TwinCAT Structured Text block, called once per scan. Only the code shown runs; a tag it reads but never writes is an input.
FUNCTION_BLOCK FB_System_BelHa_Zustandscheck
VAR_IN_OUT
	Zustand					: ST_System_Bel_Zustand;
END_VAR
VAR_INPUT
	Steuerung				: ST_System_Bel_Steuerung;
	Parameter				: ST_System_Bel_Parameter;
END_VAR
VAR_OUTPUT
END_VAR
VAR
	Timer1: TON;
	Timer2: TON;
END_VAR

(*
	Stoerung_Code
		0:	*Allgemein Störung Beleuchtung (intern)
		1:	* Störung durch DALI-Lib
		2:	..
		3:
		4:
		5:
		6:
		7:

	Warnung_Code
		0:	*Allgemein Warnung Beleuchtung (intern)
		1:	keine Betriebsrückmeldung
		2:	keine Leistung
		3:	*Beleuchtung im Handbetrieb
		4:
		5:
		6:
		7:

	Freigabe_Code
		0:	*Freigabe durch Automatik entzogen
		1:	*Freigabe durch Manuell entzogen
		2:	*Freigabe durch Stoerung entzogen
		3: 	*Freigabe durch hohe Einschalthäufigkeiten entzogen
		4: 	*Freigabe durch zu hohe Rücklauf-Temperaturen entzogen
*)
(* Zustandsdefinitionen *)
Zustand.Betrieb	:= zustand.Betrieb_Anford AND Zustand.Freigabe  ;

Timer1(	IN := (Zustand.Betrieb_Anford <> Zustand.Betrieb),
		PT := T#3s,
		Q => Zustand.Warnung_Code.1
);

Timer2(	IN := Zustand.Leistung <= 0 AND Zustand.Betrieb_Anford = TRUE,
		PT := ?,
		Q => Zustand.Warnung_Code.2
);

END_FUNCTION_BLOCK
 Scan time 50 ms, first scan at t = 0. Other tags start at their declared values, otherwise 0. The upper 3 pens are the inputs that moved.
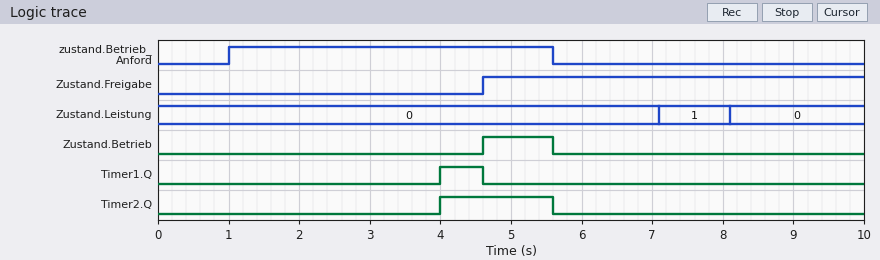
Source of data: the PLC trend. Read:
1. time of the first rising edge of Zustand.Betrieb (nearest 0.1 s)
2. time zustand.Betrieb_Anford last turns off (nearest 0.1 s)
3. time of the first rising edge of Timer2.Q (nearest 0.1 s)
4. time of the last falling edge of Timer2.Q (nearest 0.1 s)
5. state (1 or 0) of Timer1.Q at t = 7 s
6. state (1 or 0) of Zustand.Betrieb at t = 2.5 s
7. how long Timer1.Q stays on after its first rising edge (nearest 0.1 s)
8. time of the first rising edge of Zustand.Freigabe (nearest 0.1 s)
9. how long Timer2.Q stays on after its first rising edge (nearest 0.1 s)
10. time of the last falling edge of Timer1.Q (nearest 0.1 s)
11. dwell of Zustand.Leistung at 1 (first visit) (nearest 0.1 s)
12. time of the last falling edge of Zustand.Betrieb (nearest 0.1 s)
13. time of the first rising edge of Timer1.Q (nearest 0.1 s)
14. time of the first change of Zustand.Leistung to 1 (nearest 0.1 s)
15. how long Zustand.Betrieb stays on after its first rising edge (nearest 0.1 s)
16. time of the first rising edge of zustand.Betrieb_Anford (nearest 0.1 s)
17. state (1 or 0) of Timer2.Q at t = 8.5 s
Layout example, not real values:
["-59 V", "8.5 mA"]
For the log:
["4.6 s", "5.6 s", "4.0 s", "5.6 s", "0", "0", "0.6 s", "4.6 s", "1.6 s", "4.6 s", "1.0 s", "5.6 s", "4.0 s", "7.1 s", "1.0 s", "1.0 s", "0"]
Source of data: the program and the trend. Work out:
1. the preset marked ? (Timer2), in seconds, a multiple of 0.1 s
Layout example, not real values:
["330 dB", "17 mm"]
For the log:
["3.0 s"]
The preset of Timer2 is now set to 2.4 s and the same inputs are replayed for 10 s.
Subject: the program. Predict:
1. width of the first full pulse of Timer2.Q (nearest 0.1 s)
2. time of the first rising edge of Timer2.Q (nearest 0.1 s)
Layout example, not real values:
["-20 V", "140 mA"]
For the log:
["2.2 s", "3.4 s"]
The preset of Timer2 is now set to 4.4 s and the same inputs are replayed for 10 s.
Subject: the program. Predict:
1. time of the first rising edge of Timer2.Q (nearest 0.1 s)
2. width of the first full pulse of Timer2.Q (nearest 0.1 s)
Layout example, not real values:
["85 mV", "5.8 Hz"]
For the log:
["5.4 s", "0.2 s"]
